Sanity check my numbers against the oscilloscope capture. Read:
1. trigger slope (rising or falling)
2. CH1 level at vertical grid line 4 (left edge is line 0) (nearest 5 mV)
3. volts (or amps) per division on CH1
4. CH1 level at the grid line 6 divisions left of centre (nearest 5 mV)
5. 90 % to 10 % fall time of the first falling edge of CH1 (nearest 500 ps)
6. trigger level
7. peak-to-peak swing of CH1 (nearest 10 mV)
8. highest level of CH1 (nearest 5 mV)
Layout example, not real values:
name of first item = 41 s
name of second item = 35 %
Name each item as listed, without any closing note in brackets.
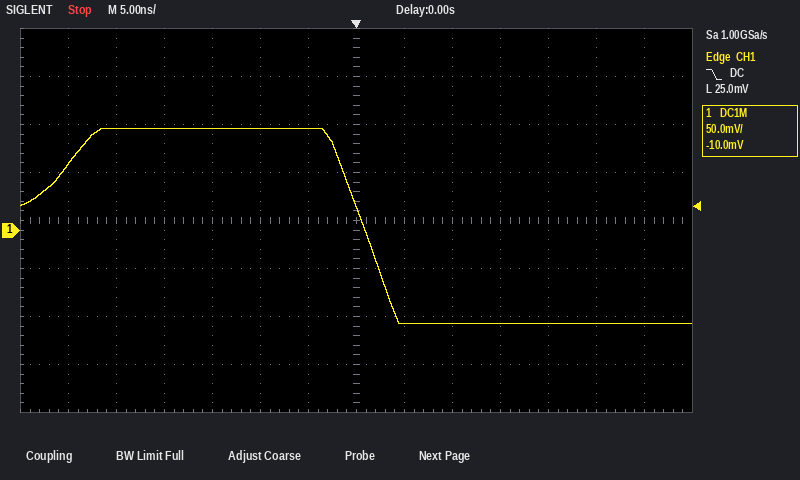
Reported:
trigger slope = falling
CH1 level at vertical grid line 4 (left edge is line 0) = 105 mV
volts (or amps) per division on CH1 = 50 mV
CH1 level at the grid line 6 divisions left of centre = 70 mV
90 % to 10 % fall time of the first falling edge of CH1 = 6.0 ns
trigger level = 25.0 mV
peak-to-peak swing of CH1 = 200 mV
highest level of CH1 = 105 mV
